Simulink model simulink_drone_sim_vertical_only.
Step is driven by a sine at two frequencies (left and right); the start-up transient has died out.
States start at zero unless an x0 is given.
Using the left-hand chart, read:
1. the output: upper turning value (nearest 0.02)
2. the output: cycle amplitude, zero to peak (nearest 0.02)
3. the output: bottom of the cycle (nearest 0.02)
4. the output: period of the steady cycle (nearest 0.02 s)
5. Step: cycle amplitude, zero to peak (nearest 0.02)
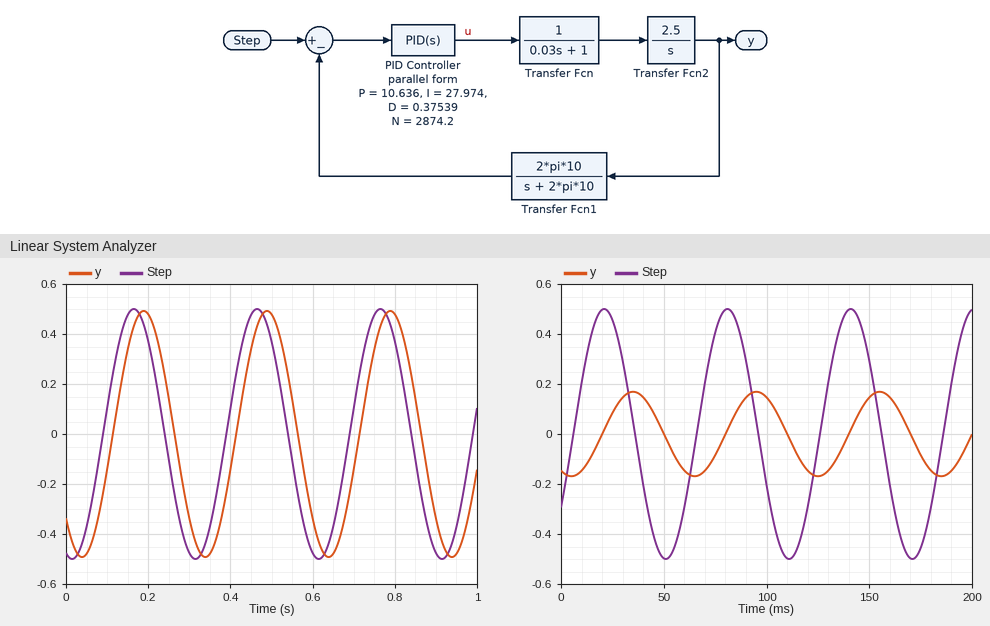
0.50
0.50
-0.50
0.30 s
0.50
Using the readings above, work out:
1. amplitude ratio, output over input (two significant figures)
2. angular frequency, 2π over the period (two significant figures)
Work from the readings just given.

1.0
21 rad/s
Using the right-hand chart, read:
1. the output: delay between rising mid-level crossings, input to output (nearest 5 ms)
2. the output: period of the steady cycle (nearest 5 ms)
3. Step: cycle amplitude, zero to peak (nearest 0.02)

15 ms
60 ms
0.50
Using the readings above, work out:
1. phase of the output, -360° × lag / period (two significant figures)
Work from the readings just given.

-90°
